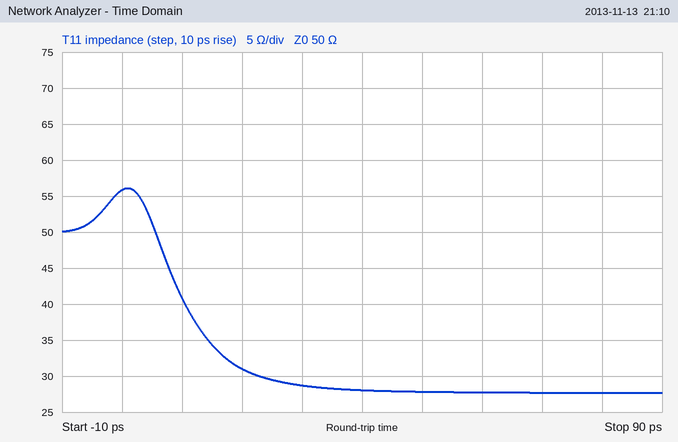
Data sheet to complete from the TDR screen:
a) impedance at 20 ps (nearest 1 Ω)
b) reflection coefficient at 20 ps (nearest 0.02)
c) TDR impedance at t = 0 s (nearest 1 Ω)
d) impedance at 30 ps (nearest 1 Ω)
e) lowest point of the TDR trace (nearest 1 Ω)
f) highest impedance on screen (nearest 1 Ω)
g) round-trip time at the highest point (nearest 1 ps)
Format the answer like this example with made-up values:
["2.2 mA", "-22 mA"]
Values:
["31 Ω", "-0.24", "56 Ω", "29 Ω", "28 Ω", "56 Ω", "1 ps"]
